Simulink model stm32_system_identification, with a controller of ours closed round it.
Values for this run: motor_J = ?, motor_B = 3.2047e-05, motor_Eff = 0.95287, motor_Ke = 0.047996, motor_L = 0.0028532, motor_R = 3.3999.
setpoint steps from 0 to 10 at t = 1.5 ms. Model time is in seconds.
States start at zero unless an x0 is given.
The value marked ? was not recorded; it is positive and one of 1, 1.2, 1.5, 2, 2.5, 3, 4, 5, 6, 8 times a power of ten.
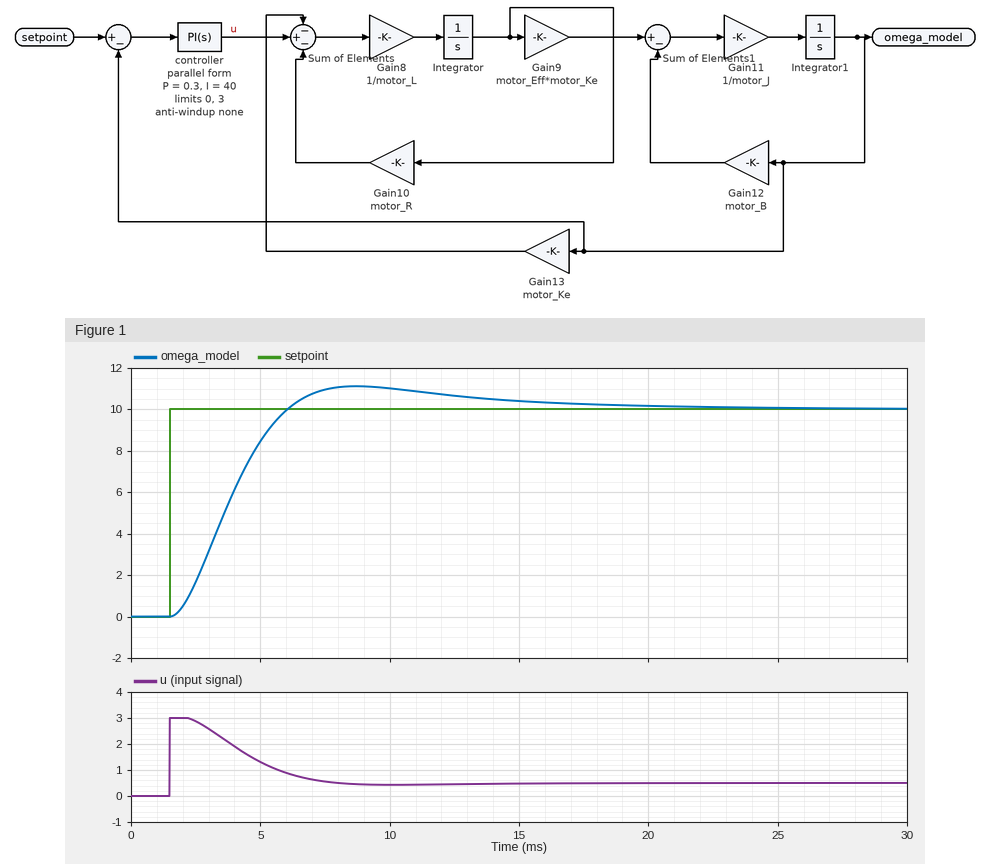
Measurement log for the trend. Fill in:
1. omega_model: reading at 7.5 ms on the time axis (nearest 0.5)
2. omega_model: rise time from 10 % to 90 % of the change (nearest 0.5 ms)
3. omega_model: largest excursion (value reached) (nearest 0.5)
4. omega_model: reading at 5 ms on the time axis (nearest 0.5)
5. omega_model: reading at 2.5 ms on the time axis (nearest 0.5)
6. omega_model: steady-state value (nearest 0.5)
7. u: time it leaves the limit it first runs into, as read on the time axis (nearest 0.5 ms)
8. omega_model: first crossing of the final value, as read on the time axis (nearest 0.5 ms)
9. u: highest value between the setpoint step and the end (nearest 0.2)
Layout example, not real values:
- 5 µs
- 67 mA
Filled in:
- 11.0
- 3.0 ms
- 11.0
- 8.5
- 1.5
- 10.0
- 2.5 ms
- 6.0 ms
- 3.0
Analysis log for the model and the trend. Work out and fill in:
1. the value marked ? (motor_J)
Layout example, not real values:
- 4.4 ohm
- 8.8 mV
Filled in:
- 1e-05
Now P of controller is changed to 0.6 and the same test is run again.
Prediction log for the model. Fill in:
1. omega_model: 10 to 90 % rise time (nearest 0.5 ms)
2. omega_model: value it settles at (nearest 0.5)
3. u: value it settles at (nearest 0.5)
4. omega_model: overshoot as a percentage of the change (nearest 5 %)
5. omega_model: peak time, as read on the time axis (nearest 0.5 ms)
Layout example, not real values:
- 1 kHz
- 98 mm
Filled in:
- 2.5 ms
- 10.0
- 0.5
- 10 %
- 6.5 ms
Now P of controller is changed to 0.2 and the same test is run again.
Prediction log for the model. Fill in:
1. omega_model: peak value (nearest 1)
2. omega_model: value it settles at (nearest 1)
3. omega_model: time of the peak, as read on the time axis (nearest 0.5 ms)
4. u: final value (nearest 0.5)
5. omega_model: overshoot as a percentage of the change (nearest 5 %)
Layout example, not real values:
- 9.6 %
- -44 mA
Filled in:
- 12
- 10
- 11.0 ms
- 0.5
- 20 %
